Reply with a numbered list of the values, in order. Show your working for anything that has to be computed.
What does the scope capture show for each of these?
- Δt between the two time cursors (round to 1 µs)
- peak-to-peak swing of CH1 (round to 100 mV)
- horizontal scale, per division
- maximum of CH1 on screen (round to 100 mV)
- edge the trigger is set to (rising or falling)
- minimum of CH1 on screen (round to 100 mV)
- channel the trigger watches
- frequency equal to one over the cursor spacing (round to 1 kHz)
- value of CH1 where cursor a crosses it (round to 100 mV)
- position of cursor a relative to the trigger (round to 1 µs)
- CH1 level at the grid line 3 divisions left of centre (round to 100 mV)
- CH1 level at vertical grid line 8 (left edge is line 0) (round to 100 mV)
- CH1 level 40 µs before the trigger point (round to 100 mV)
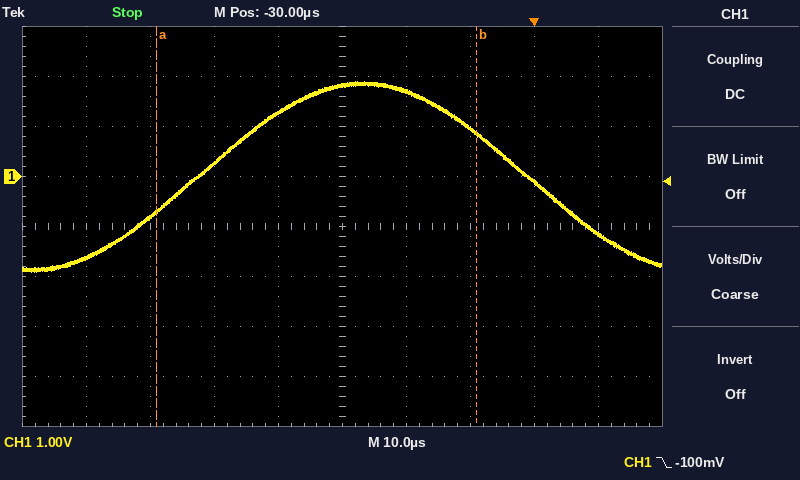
1. 50 µs
2. 1.9 V − (-1.9 V) = 3.8 V
3. 10 µs
4. 1.9 V
5. falling
6. -1.9 V
7. CH1
8. 1 / 50 µs ≈ 20 kHz
9. -700 mV
10. -59 µs
11. -800 mV
12. -100 mV
13. 1.3 V
